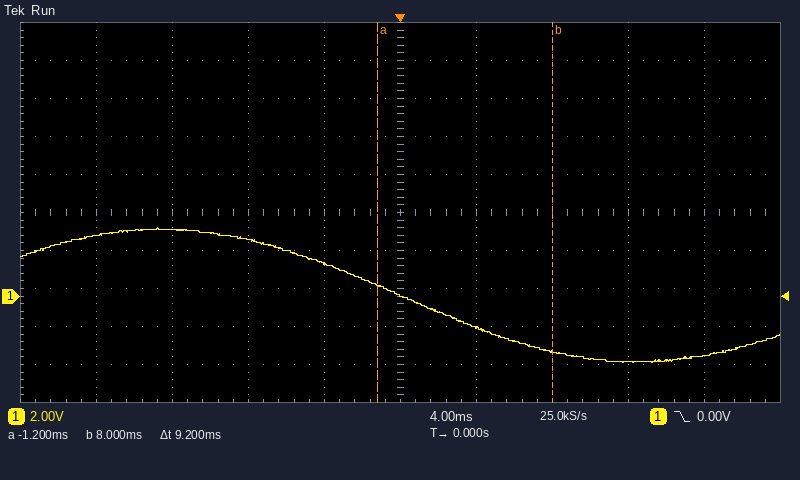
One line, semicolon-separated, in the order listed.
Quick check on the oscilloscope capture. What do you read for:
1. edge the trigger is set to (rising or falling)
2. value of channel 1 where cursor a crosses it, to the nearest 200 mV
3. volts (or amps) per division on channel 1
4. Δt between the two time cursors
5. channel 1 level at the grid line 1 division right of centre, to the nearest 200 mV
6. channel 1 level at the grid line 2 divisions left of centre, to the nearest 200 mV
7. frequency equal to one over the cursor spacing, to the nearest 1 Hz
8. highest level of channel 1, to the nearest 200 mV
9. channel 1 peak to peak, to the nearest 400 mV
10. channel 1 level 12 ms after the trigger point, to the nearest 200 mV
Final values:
falling; 600 mV; 2 V; 9.2 ms; -1.6 V; 3.0 V; 109 Hz; 3.6 V; 7.2 V; -3.4 V
